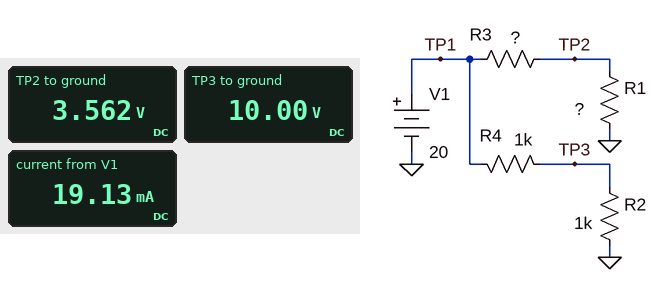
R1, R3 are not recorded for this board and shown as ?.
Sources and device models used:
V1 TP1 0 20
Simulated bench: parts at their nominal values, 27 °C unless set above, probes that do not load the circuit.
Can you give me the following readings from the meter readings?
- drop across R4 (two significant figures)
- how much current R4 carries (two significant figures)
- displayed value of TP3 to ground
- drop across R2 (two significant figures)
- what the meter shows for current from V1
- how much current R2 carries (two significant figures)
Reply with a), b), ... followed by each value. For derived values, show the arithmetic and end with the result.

a) 20 V - 10 V = 10 V
b) (20 V - 10 V) / 1 kΩ = 10 mA
c) 10.00 V
d) 10 V = 10 V
e) 19.13 mA
f) (10 V) / 1 kΩ = 10 mA
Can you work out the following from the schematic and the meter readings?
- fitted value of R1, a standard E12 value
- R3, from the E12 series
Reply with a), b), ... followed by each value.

a) 390 Ω
b) 1.8 kΩ
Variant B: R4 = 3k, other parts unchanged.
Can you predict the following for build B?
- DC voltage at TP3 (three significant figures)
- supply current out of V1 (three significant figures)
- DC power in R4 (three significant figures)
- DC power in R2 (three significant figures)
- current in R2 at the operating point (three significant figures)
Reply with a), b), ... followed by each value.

a) 5.00 V
b) 14.1 mA
c) 75.0 mW
d) 25.0 mW
e) 5.00 mA
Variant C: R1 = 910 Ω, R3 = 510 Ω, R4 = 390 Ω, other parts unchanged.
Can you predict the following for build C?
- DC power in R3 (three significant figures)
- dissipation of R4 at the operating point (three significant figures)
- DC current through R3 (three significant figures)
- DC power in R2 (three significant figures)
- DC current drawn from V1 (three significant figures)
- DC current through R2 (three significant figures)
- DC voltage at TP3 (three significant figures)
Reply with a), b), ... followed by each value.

a) 101 mW
b) 80.7 mW
c) 14.1 mA
d) 207 mW
e) 28.5 mA
f) 14.4 mA
g) 14.4 V
